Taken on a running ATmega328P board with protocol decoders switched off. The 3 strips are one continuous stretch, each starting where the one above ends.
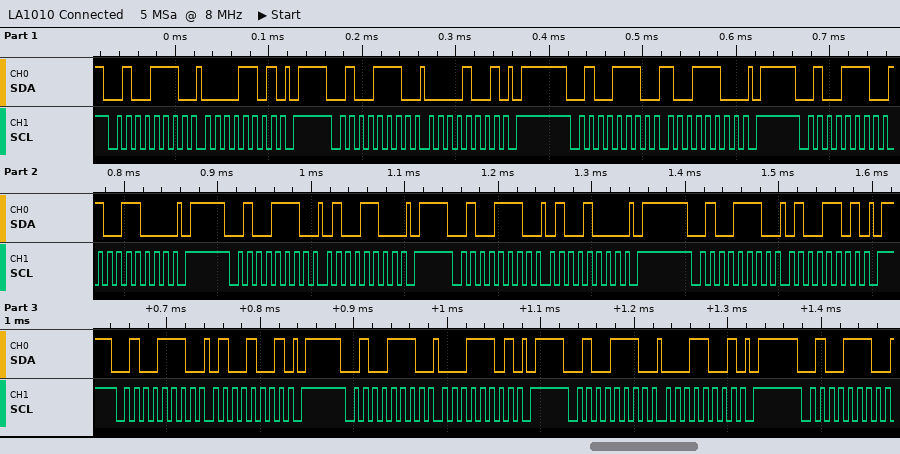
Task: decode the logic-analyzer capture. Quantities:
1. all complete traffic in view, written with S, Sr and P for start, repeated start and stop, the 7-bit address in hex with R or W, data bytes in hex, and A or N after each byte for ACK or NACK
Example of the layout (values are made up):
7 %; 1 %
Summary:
S 27W A 0D A P S 27W A 09 A P S 27W A 9C A P S 27W A 98 A P S 27W A 4C A P S 27W A 48 A P S 27W A 4D A P S 27W A 49 A P S 27W A 1D A P S 27W A 19 A P S 27W A
